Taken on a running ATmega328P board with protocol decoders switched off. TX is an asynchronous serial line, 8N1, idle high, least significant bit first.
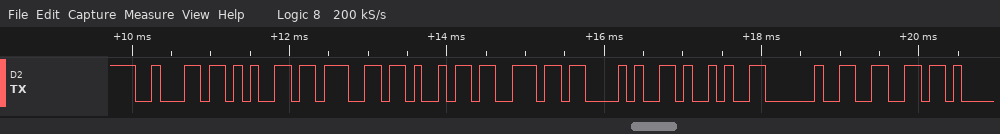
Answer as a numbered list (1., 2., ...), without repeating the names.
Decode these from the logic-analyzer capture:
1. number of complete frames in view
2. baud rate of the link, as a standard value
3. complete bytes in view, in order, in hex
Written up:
1. 9
2. 9600 baud
3. 0x62 0x65 0x67 0x69 0x6E 0x28 0x29 0x20 0x66
